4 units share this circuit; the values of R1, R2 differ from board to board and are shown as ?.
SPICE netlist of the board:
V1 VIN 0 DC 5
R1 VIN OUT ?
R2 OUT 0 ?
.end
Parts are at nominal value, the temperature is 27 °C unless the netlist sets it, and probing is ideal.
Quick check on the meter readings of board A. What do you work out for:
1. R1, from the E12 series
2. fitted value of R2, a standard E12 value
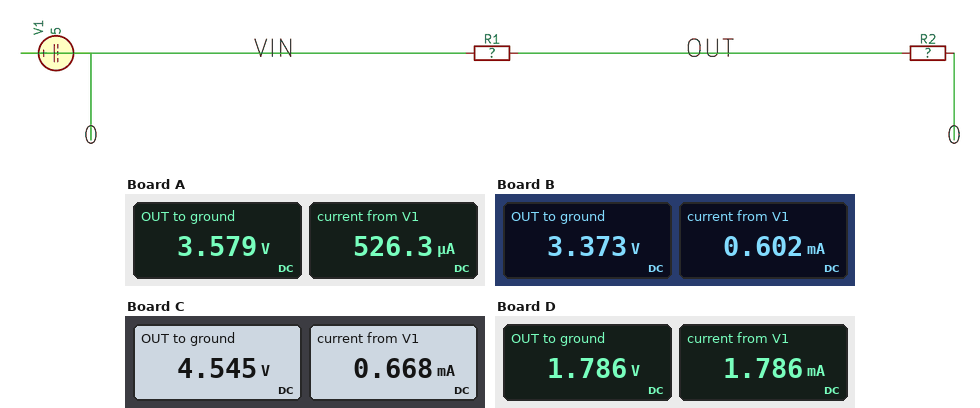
2.7 kΩ
6.8 kΩ
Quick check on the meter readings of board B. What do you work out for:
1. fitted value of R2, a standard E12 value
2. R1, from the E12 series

5.6 kΩ
2.7 kΩ
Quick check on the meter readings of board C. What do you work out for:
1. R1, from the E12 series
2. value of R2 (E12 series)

680 Ω
6.8 kΩ
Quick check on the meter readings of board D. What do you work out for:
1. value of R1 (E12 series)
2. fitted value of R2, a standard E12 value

1.8 kΩ
1 kΩ
